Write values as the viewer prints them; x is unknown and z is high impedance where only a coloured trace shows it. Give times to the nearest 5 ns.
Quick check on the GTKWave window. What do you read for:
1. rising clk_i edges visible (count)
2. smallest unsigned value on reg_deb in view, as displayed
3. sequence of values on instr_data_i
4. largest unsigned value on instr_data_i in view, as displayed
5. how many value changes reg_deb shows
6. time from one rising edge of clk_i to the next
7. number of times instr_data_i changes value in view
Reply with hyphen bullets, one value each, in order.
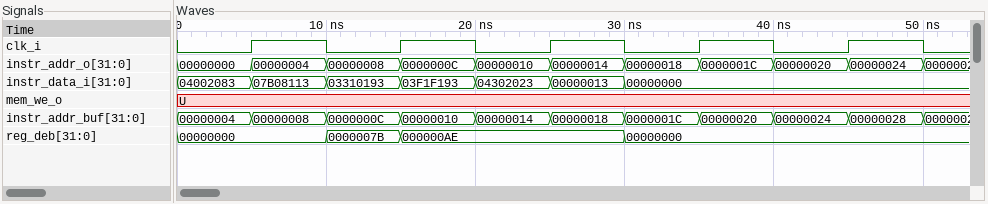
- 5
- 00000000
- 04002083, 07B08113, 03310193, 03F1F193, 04302023, 00000013, 00000000
- 07B08113
- 3
- 10 ns
- 6
